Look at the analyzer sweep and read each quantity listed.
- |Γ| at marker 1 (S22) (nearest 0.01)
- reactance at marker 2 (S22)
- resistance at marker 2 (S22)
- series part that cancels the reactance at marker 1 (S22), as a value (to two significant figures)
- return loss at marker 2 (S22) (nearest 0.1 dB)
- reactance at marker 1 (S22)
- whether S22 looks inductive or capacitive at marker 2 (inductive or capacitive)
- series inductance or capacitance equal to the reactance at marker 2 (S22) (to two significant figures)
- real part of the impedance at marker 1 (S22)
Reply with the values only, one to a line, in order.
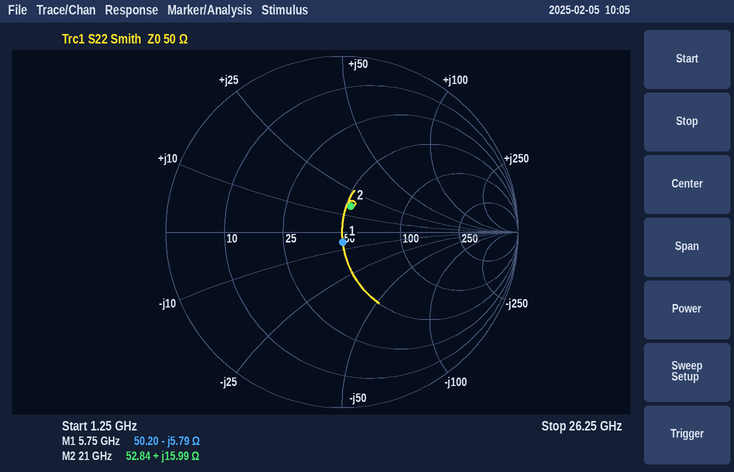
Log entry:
0.06
+15.99 Ω
52.84 Ω
160 pH
16.1 dB
-5.79 Ω
inductive
120 pH
50.20 Ω
